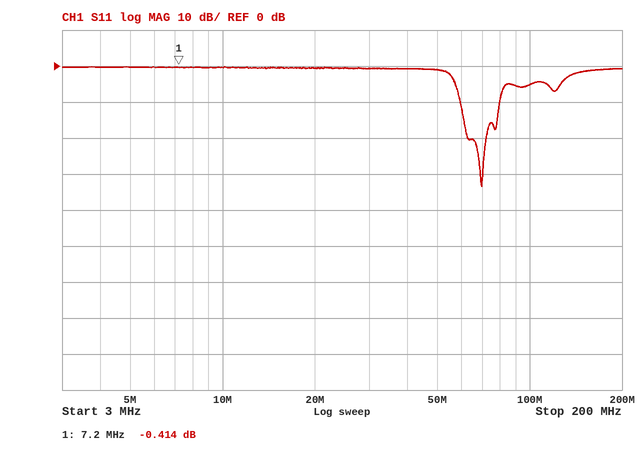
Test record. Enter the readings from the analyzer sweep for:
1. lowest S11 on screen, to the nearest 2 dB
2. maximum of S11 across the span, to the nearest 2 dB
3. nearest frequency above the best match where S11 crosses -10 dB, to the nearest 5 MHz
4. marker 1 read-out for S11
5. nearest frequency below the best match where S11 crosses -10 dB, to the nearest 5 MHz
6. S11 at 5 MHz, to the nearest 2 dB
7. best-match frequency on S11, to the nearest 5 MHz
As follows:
-34 dB
0 dB
80 MHz
-0.414 dB
60 MHz
0 dB
70 MHz
